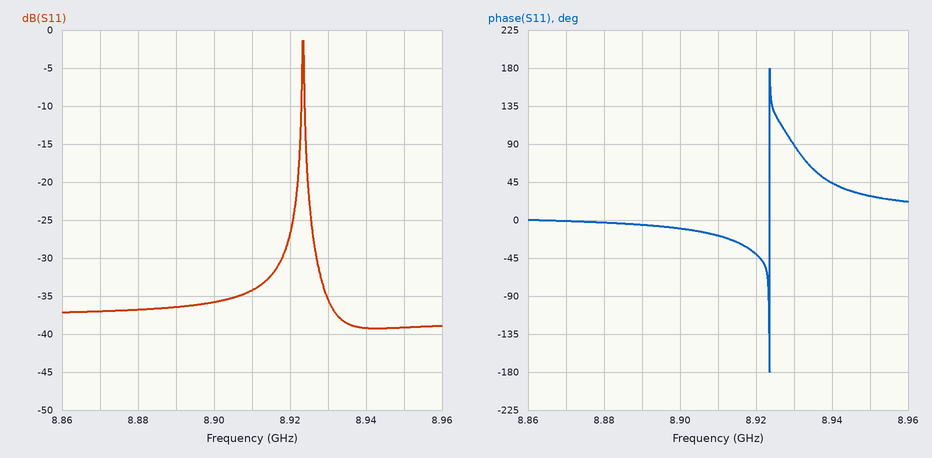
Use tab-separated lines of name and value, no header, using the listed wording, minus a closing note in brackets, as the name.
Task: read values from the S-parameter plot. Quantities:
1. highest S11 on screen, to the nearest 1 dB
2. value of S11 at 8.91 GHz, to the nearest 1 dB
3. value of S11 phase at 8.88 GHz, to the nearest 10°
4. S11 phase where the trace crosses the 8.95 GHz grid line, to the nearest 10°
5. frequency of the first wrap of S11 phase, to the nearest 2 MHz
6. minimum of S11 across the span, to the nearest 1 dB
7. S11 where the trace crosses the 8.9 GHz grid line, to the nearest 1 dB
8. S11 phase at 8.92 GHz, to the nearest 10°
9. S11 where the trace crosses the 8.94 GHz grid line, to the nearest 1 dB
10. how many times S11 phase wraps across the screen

highest S11 on screen, to the nearest 1 dB	-1 dB
value of S11 at 8.91 GHz, to the nearest 1 dB	-34 dB
value of S11 phase at 8.88 GHz, to the nearest 10°	0°
S11 phase where the trace crosses the 8.95 GHz grid line, to the nearest 10°	30°
frequency of the first wrap of S11 phase, to the nearest 2 MHz	8.924 GHz
minimum of S11 across the span, to the nearest 1 dB	-39 dB
S11 where the trace crosses the 8.9 GHz grid line, to the nearest 1 dB	-36 dB
S11 phase at 8.92 GHz, to the nearest 10°	-40°
S11 where the trace crosses the 8.94 GHz grid line, to the nearest 1 dB	-39 dB
how many times S11 phase wraps across the screen	1
